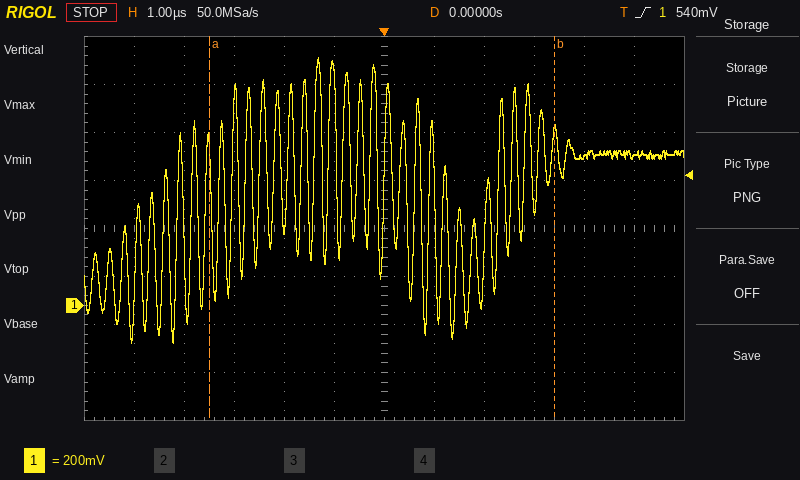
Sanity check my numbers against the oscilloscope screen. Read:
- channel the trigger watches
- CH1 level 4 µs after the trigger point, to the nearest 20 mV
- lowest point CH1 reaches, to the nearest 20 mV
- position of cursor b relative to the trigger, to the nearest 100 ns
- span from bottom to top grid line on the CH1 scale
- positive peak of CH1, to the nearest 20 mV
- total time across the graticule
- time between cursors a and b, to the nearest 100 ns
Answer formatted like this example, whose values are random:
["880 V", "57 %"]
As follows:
["CH1", "620 mV", "-160 mV", "+3.4 µs", "1.6 V", "1.04 V", "12 µs", "6.9 µs"]
